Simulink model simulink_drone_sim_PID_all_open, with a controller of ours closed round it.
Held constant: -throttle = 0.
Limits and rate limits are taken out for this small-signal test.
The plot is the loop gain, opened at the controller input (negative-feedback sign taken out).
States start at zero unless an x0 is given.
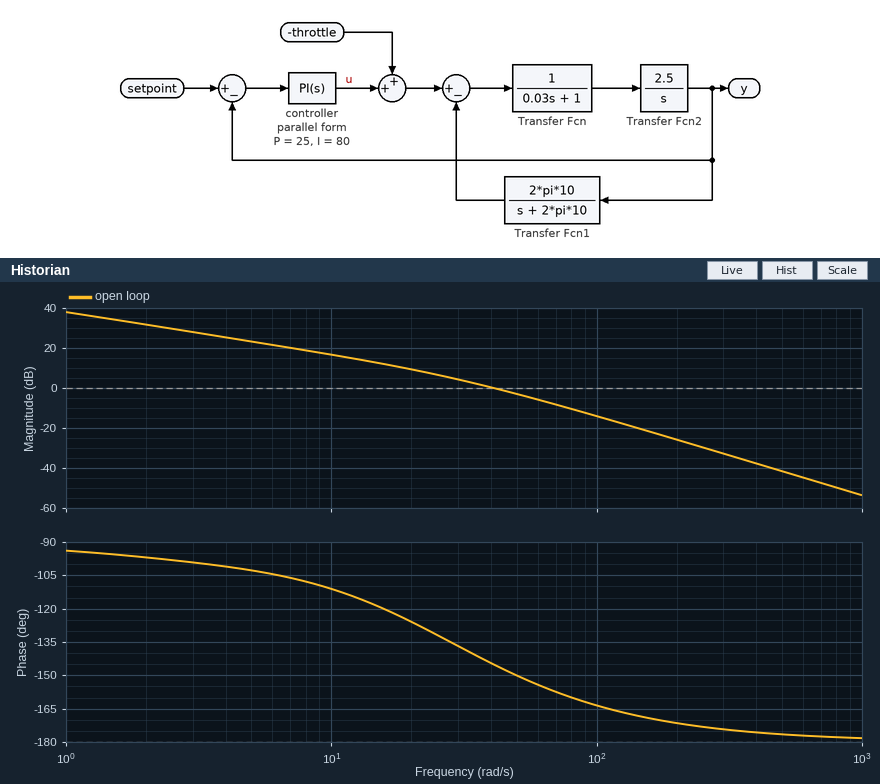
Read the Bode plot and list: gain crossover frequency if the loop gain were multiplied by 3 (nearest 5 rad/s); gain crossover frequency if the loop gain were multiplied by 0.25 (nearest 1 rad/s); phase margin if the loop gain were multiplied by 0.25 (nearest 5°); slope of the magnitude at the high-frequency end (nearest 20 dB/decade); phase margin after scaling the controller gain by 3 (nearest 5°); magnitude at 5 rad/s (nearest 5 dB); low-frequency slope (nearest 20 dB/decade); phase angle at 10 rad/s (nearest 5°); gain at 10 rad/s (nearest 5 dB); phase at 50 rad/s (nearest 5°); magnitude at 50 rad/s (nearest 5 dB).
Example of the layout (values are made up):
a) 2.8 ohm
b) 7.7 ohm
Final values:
a) 75 rad/s
b) 16 rad/s
c) 60°
d) -40 dB/decade
e) 20°
f) 25 dB
g) -20 dB/decade
h) -110°
i) 15 dB
j) -150°
k) -5 dB
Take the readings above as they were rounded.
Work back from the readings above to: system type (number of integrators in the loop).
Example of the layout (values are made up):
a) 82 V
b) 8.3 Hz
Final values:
a) 1
